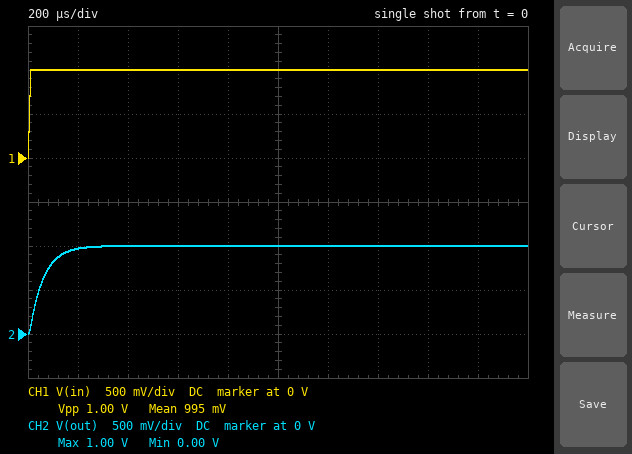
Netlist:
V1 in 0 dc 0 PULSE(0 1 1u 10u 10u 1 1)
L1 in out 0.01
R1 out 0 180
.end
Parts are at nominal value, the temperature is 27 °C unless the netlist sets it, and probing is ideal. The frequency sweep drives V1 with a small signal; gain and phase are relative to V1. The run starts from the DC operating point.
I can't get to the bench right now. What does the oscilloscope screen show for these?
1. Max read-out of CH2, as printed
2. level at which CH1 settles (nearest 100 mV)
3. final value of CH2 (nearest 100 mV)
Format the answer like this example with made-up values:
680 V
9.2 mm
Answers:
1.00 V
1.0 V
1.0 V
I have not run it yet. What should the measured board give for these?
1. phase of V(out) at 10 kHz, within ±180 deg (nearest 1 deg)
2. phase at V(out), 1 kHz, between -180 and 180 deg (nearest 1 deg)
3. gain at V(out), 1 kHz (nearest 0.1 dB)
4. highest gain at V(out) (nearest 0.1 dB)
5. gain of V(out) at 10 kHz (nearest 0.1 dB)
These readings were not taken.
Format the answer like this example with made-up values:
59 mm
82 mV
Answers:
-74 deg
-19 deg
-0.5 dB
0 dB
-11.2 dB
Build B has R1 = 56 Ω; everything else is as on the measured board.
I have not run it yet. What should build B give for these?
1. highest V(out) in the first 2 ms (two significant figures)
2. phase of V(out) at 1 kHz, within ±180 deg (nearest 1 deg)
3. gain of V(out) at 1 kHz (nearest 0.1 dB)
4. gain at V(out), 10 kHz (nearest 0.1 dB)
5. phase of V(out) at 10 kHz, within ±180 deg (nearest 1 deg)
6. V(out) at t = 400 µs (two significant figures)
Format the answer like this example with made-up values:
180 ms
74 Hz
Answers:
1.0 V
-48 deg
-3.5 dB
-21.0 dB
-85 deg
890 mV
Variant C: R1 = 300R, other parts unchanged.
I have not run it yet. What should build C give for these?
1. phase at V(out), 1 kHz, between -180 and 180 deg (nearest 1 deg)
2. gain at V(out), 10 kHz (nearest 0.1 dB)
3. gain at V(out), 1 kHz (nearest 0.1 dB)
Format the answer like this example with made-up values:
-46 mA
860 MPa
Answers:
-12 deg
-7.3 dB
-0.2 dB
